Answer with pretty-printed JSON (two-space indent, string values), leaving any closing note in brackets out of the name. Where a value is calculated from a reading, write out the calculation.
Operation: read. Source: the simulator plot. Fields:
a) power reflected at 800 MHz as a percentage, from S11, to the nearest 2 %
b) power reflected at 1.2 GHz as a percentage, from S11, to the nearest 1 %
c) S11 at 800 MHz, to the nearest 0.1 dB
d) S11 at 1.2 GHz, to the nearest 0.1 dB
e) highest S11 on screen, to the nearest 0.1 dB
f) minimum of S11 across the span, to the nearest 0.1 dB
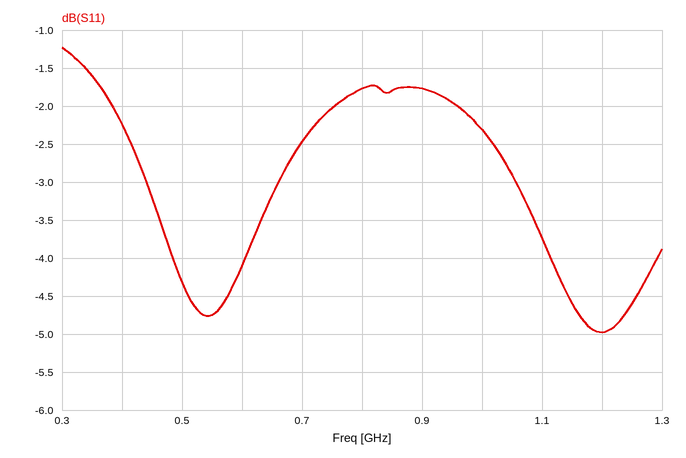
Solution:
{
  "power reflected at 800 MHz as a percentage, from S11, to the nearest 2 %": "10^(-1.8/10) ≈ 66 %",
  "power reflected at 1.2 GHz as a percentage, from S11, to the nearest 1 %": "10^(-5/10) ≈ 32 %",
  "S11 at 800 MHz, to the nearest 0.1 dB": "-1.8 dB",
  "S11 at 1.2 GHz, to the nearest 0.1 dB": "-5.0 dB",
  "highest S11 on screen, to the nearest 0.1 dB": "-1.2 dB",
  "minimum of S11 across the span, to the nearest 0.1 dB": "-5.0 dB"
}
